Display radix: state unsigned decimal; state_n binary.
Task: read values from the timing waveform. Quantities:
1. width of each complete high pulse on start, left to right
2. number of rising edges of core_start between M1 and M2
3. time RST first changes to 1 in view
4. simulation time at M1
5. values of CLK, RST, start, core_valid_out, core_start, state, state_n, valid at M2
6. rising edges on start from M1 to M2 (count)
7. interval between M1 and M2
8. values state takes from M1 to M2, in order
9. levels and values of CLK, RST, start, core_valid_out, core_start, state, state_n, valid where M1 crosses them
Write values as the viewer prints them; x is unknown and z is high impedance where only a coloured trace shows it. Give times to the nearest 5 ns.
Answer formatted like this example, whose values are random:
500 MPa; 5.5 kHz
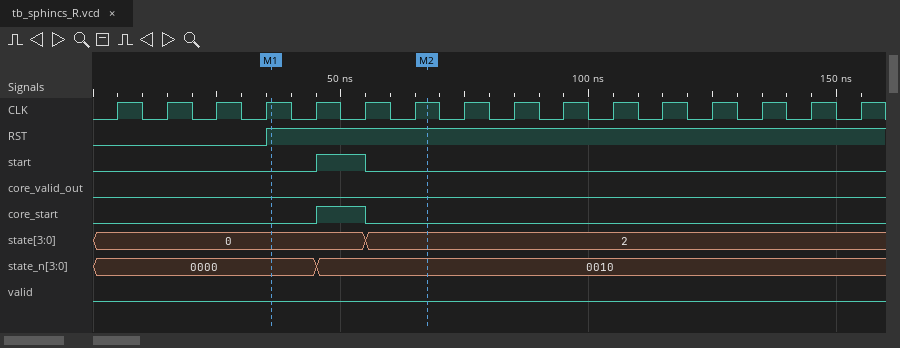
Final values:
10 ns; 1; 35 ns; 35 ns; CLK=1, RST=1, start=0, core_valid_out=0, core_start=0, state=2, state_n=0010, valid=0; 1; 30 ns; 0, 2; CLK=1, RST=1, start=0, core_valid_out=0, core_start=0, state=0, state_n=0000, valid=0
